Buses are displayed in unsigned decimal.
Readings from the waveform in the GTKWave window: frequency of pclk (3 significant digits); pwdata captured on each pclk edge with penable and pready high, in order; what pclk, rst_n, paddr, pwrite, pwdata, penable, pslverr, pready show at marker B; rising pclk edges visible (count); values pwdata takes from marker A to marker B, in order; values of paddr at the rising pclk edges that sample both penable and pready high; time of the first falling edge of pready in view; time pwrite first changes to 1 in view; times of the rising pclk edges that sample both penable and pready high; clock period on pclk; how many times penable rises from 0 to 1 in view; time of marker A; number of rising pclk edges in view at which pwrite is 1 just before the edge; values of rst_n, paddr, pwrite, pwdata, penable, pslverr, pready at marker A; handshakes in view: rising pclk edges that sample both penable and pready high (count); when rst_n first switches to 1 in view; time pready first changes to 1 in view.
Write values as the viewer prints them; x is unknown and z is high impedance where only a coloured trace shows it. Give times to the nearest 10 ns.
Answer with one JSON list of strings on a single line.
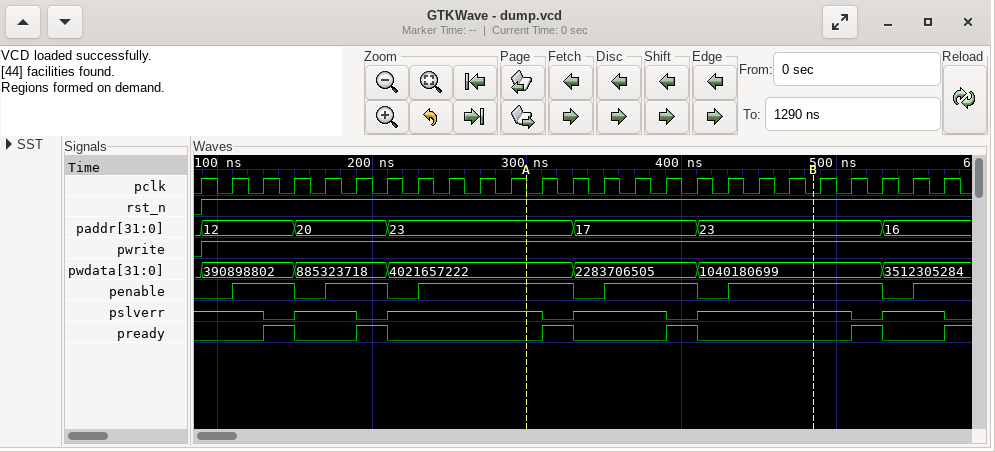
["50.0 MHz", "390898802, 885323718, 4021657222, 2283706505, 1040180699", "pclk=0, rst_n=1, paddr=23, pwrite=1, pwdata=1040180699, penable=1, pslverr=z, pready=0", "25", "4021657222, 2283706505, 1040180699", "12, 20, 23, 17, 23", "150 ns", "90 ns", "150 ns, 210 ns, 330 ns, 410 ns, 530 ns", "20 ns", "6", "300 ns", "24", "rst_n=1, paddr=23, pwrite=1, pwdata=4021657222, penable=1, pslverr=z, pready=0", "5", "90 ns", "130 ns"]
